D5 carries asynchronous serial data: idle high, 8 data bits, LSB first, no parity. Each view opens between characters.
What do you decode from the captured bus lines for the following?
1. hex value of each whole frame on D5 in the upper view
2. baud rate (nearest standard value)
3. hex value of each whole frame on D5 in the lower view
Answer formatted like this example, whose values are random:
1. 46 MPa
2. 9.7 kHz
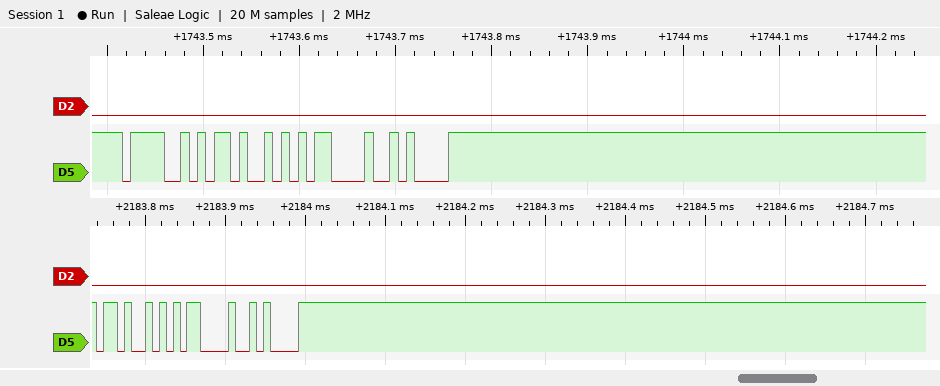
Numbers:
1. 4F, 4B, 0D, 0A
2. 115200 baud
3. 4B, 0D, 0A
